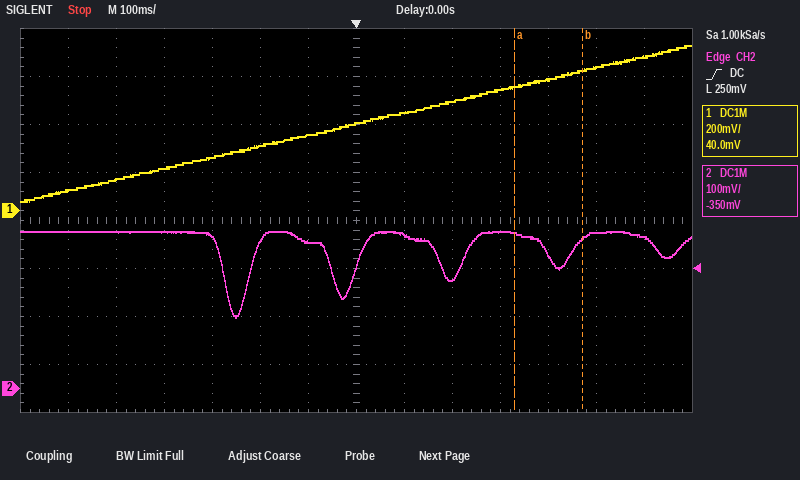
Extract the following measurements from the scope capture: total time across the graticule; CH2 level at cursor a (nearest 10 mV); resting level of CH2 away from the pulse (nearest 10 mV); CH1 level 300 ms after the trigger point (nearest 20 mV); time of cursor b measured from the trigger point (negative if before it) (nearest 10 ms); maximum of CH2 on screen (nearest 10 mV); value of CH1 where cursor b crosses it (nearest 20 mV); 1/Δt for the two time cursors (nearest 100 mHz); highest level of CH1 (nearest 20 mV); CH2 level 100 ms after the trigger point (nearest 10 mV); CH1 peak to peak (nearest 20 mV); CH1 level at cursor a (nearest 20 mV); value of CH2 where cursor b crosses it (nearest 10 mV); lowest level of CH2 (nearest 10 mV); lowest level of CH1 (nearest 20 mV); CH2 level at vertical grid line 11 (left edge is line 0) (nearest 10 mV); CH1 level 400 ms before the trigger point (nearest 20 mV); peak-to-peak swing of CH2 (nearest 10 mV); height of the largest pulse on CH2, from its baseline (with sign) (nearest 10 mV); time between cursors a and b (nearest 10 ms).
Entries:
1.4 s
320 mV
330 mV
500 mV
+470 ms
330 mV
580 mV
7.1 Hz
680 mV
320 mV
640 mV
520 mV
310 mV
150 mV
40 mV
280 mV
180 mV
180 mV
-180 mV
140 ms
